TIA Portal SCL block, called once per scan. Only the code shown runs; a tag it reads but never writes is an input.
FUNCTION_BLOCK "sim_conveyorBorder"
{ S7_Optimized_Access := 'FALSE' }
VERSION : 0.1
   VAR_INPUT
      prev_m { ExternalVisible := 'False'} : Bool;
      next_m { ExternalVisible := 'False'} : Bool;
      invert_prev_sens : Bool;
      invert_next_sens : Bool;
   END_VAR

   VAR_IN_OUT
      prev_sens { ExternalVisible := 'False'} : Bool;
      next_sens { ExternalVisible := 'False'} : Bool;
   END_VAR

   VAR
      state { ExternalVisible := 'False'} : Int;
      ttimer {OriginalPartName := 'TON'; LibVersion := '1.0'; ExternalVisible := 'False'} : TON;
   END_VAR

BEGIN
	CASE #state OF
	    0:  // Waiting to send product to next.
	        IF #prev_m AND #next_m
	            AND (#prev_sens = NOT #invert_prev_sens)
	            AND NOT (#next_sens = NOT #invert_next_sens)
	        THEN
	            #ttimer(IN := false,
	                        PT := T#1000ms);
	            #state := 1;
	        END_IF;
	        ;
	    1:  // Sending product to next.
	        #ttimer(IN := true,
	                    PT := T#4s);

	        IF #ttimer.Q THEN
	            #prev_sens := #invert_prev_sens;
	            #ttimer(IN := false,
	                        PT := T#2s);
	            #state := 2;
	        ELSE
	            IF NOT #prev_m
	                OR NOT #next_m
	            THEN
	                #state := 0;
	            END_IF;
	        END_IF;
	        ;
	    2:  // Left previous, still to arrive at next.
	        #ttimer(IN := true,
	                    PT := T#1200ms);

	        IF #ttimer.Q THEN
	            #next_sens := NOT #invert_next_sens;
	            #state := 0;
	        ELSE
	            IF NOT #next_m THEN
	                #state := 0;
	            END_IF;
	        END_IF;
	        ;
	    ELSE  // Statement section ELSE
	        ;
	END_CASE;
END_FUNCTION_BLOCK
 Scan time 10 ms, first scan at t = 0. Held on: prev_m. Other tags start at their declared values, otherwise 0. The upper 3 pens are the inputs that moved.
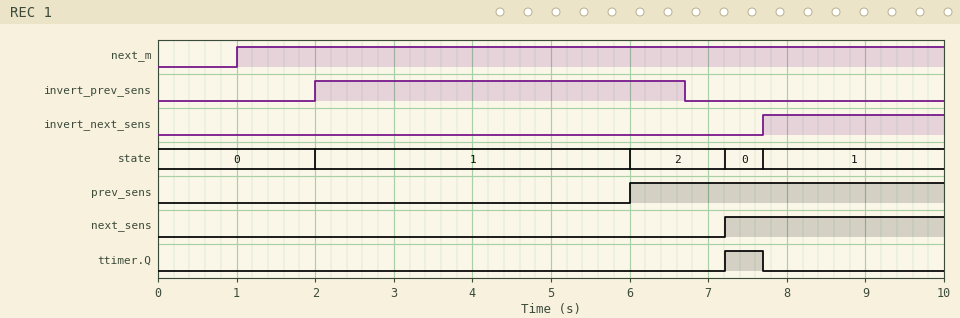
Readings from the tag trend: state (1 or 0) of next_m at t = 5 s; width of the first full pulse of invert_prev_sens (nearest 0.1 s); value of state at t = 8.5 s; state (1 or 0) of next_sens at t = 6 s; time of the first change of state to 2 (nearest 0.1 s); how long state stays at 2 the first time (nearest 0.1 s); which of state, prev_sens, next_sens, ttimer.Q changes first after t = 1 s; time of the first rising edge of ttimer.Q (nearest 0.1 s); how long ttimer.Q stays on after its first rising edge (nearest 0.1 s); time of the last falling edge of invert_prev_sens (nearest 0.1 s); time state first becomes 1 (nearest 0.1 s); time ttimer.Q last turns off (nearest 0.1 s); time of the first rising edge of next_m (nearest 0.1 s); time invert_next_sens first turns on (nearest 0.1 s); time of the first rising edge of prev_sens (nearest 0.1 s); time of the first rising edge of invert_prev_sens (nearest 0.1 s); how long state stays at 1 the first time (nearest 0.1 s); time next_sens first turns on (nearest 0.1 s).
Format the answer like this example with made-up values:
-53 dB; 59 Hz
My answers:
1; 4.7 s; 1; 0; 6.0 s; 1.2 s; state; 7.2 s; 0.5 s; 6.7 s; 2.0 s; 7.7 s; 1.0 s; 7.7 s; 6.0 s; 2.0 s; 4.0 s; 7.2 s
